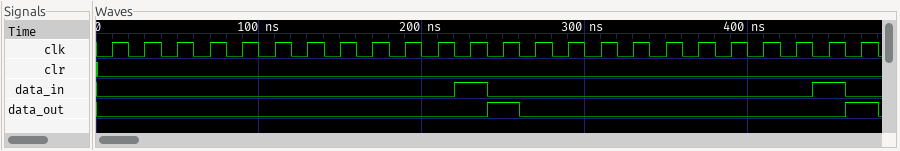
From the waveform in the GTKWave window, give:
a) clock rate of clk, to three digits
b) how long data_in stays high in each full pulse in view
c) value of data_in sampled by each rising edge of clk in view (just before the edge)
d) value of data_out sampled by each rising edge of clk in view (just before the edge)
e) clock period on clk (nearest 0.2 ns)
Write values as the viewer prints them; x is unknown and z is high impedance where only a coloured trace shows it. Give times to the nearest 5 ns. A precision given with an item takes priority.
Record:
50.0 MHz
20 ns, 20 ns
0 0 0 0 0 0 0 0 0 0 0 1 0 0 0 0 0 0 0 0 0 0 1 0
0 0 0 0 0 0 0 0 0 0 0 0 1 0 0 0 0 0 0 0 0 0 0 1
20 ns
